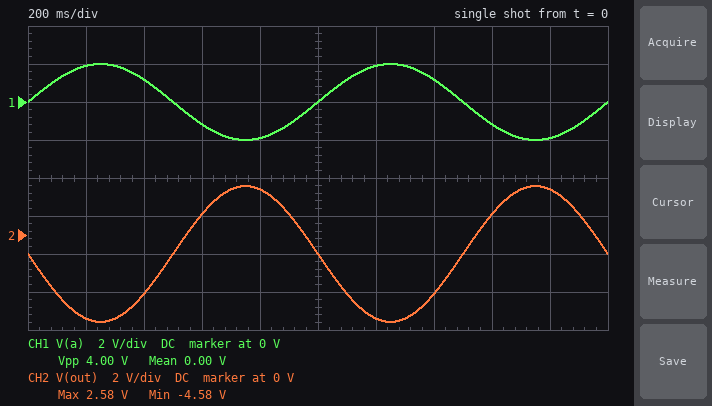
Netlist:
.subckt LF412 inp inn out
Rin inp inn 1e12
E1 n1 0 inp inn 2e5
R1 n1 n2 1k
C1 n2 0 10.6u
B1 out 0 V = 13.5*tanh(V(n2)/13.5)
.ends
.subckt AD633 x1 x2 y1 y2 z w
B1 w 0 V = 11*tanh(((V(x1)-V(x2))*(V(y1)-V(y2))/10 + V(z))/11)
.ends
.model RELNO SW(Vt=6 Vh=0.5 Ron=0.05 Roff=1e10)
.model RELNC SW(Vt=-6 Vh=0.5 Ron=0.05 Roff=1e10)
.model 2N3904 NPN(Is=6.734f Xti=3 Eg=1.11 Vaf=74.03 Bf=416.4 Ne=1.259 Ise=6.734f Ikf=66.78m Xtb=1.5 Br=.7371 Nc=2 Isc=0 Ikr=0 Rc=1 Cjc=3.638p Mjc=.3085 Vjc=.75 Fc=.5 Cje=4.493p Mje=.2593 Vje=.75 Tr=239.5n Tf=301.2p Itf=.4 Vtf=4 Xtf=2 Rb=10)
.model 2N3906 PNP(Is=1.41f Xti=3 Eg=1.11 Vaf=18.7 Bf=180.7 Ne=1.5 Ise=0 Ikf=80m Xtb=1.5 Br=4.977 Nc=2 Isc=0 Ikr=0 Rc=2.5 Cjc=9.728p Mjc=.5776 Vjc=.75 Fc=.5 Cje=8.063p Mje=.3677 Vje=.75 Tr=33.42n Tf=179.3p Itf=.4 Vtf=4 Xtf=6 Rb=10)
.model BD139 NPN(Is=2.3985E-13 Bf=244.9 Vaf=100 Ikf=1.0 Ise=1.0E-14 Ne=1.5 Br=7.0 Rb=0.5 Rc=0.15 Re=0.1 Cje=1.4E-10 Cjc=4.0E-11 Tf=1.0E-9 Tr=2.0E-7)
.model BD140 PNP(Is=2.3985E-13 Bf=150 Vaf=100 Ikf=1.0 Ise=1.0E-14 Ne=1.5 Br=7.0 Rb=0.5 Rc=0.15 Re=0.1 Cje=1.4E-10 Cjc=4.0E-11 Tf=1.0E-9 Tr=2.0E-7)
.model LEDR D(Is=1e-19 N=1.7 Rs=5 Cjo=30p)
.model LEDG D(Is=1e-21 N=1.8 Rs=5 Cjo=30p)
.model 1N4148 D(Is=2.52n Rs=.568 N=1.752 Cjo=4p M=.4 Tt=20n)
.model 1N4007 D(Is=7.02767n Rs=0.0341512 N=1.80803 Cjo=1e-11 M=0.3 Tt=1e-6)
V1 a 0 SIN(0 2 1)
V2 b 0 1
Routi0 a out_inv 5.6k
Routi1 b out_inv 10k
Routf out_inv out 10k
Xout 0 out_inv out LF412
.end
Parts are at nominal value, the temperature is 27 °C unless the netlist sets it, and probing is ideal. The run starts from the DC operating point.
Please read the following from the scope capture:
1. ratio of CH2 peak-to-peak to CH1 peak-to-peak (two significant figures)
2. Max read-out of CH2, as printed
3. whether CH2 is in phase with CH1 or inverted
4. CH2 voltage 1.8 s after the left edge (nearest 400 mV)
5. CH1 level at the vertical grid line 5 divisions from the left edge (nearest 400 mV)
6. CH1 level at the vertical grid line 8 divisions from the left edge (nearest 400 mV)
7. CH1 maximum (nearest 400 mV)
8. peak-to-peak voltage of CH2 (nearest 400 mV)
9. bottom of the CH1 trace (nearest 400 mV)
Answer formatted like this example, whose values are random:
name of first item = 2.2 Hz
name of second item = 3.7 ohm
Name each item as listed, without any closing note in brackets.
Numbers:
ratio of CH2 peak-to-peak to CH1 peak-to-peak = 1.8
Max read-out of CH2, as printed = 2.58 V
whether CH2 is in phase with CH1 or inverted = inverted
CH2 voltage 1.8 s after the left edge = 2.4 V
CH1 level at the vertical grid line 5 divisions from the left edge = 0 V
CH1 level at the vertical grid line 8 divisions from the left edge = -1.2 V
CH1 maximum = 2.0 V
peak-to-peak voltage of CH2 = 7.2 V
bottom of the CH1 trace = -2.0 V
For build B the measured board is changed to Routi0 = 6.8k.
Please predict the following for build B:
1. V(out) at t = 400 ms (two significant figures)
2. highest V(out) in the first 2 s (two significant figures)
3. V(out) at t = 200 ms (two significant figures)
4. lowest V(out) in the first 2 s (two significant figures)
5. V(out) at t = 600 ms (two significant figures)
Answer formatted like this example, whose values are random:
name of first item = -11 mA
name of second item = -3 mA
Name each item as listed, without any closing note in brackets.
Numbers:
V(out) at t = 400 ms = -2.7 V
highest V(out) in the first 2 s = 1.9 V
V(out) at t = 200 ms = -3.8 V
lowest V(out) in the first 2 s = -3.9 V
V(out) at t = 600 ms = 730 mV
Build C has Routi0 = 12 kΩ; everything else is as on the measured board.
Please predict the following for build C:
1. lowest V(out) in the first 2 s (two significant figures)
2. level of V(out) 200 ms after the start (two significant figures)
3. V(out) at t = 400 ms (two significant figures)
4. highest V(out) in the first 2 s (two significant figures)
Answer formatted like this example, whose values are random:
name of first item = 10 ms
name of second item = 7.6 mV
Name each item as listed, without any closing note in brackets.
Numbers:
lowest V(out) in the first 2 s = -2.7 V
level of V(out) 200 ms after the start = -2.6 V
V(out) at t = 400 ms = -2.0 V
highest V(out) in the first 2 s = 670 mV
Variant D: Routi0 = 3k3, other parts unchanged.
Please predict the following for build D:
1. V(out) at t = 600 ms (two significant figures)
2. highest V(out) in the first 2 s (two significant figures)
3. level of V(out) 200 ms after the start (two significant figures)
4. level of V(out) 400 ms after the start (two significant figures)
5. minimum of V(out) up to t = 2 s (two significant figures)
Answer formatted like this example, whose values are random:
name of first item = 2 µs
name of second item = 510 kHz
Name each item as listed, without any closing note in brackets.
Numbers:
V(out) at t = 600 ms = 2.6 V
highest V(out) in the first 2 s = 5.1 V
level of V(out) 200 ms after the start = -6.8 V
level of V(out) 400 ms after the start = -4.6 V
minimum of V(out) up to t = 2 s = -7.1 V
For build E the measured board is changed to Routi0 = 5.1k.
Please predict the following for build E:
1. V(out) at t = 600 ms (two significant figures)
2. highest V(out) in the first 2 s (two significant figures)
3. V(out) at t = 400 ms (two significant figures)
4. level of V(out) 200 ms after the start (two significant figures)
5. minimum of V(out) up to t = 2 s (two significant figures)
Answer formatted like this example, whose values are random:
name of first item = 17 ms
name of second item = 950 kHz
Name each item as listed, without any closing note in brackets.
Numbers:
V(out) at t = 600 ms = 1.3 V
highest V(out) in the first 2 s = 2.9 V
V(out) at t = 400 ms = -3.3 V
level of V(out) 200 ms after the start = -4.7 V
minimum of V(out) up to t = 2 s = -4.9 V
